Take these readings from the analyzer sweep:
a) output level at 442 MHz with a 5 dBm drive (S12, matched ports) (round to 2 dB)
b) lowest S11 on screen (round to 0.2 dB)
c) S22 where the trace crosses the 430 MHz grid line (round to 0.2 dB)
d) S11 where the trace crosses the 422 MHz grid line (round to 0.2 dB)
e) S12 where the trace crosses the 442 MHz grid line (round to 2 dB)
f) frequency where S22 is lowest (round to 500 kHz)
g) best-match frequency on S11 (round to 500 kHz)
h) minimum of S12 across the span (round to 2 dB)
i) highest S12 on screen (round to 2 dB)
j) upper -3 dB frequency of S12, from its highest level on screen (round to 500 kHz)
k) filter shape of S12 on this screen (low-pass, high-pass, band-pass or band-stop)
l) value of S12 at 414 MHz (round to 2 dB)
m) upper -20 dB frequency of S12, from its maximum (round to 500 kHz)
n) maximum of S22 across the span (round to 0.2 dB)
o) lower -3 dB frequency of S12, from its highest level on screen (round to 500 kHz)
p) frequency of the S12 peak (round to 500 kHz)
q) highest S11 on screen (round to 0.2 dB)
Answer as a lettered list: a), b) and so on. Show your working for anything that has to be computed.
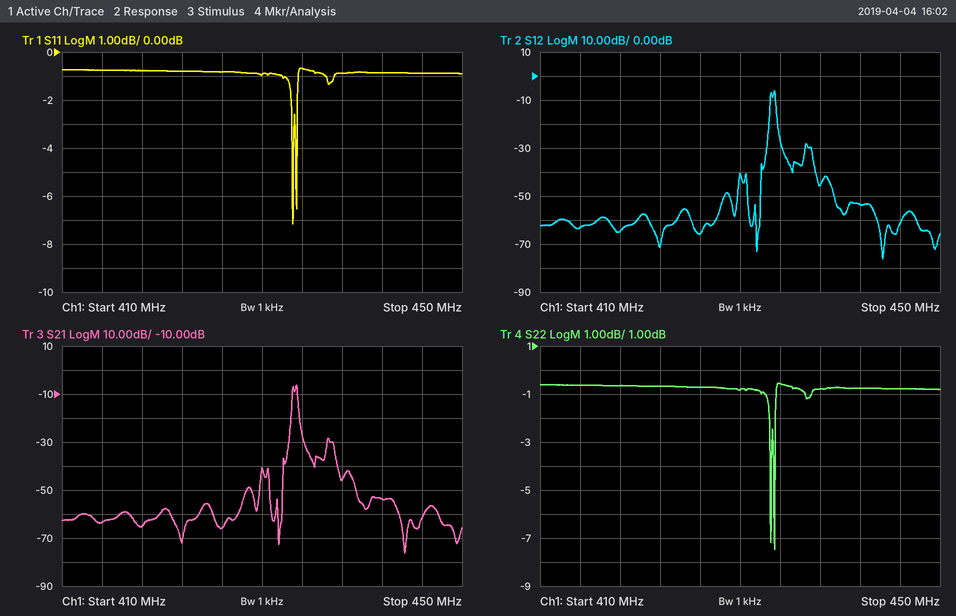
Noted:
a) 5 dBm + (-54 dB) = -48 dBm
b) -7.2 dB
c) -0.8 dB
d) -0.8 dB
e) -54 dB
f) 433.5 MHz
g) 433.0 MHz
h) -76 dB
i) -6 dB
j) 433.5 MHz
k) band-pass
l) -64 dB
m) 434.0 MHz
n) -0.6 dB
o) 433.0 MHz
p) 433.5 MHz
q) -0.6 dB
